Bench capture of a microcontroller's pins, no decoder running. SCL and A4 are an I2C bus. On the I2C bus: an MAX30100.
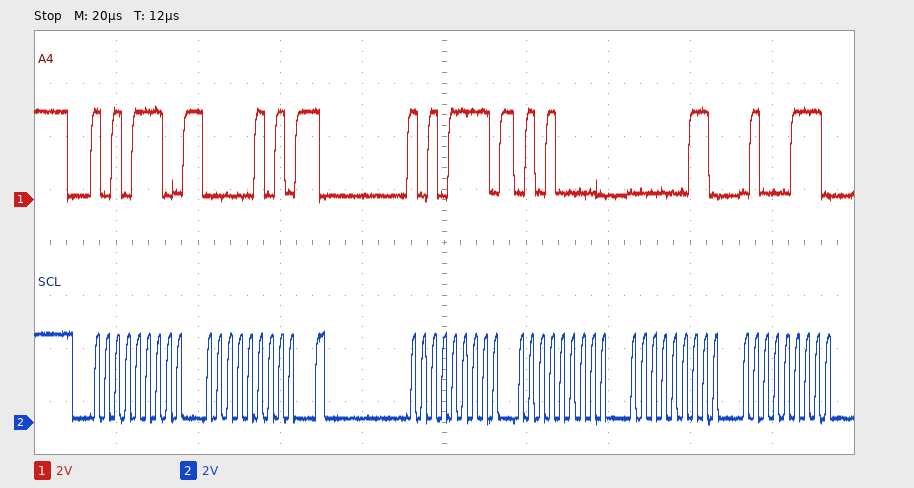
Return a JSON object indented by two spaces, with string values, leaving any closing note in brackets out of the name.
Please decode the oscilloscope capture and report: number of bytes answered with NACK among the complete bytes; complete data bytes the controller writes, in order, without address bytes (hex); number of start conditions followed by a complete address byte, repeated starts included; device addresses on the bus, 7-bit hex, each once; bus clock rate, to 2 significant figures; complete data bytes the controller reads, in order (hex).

{
  "number of bytes answered with NACK among the complete bytes": "0",
  "complete data bytes the controller writes, in order, without address bytes": "05",
  "number of start conditions followed by a complete address byte, repeated starts included": "2",
  "device addresses on the bus, 7-bit hex, each once": "0x57",
  "bus clock rate, to 2 significant figures": "400 kHz",
  "complete data bytes the controller reads, in order": "50 03 47"
}
